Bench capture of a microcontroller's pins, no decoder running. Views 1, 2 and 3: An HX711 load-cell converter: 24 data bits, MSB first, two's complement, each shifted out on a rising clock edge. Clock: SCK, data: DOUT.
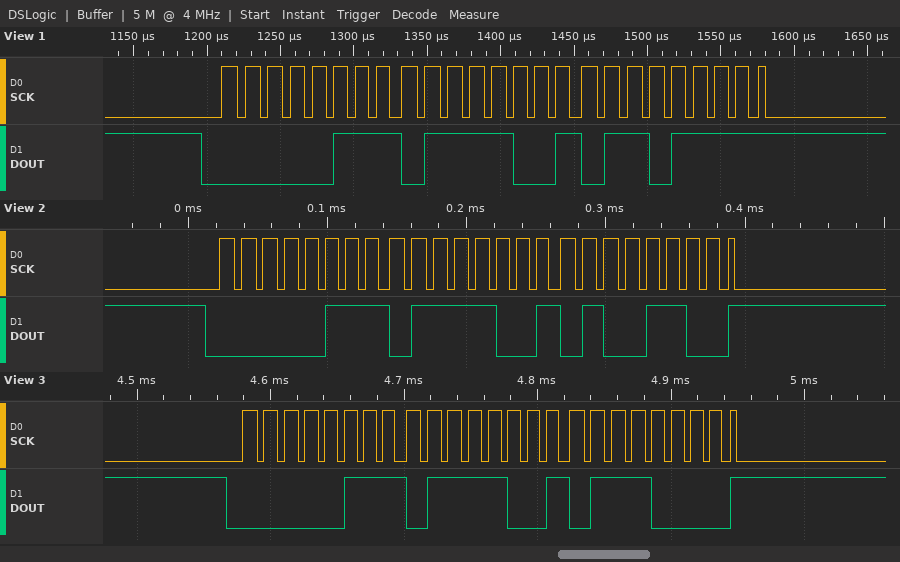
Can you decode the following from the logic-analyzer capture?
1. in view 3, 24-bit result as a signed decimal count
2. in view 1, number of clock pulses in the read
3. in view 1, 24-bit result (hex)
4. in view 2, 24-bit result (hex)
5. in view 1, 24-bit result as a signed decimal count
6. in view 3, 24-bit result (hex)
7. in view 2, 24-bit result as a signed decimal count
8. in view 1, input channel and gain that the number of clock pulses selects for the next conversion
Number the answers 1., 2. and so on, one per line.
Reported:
1. 489840
2. 25
3. 0x07796F
4. 0x07794C
5. 489839
6. 0x077970
7. 489804
8. channel A, gain 128
